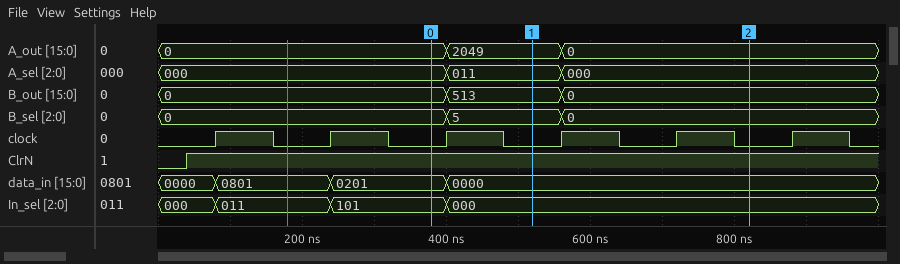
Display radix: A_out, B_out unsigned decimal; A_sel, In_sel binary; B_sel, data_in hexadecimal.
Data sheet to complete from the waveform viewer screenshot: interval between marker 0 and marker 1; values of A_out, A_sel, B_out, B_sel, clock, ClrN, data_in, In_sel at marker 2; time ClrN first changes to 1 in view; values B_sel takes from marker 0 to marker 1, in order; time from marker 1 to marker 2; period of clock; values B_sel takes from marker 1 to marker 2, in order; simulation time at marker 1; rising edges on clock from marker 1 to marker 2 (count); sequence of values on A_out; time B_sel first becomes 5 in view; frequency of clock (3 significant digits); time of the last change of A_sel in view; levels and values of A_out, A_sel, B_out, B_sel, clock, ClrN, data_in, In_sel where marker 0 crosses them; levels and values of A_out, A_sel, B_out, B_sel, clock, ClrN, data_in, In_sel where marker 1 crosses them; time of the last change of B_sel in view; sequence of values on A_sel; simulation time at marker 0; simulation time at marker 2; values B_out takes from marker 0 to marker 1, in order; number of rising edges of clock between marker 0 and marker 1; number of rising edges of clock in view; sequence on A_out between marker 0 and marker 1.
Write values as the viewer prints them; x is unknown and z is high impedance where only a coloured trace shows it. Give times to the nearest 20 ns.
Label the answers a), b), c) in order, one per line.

a) 140 ns
b) A_out=0, A_sel=000, B_out=0, B_sel=0, clock=0, ClrN=1, data_in=0000, In_sel=000
c) 40 ns
d) 0, 5
e) 300 ns
f) 160 ns
g) 5, 0
h) 520 ns
i) 2
j) 0, 2049, 0
k) 400 ns
l) 6.25 MHz
m) 560 ns
n) A_out=0, A_sel=000, B_out=0, B_sel=0, clock=0, ClrN=1, data_in=0201, In_sel=101
o) A_out=2049, A_sel=011, B_out=513, B_sel=5, clock=0, ClrN=1, data_in=0000, In_sel=000
p) 560 ns
q) 000, 011, 000
r) 380 ns
s) 820 ns
t) 0, 513
u) 1
v) 6
w) 0, 2049
